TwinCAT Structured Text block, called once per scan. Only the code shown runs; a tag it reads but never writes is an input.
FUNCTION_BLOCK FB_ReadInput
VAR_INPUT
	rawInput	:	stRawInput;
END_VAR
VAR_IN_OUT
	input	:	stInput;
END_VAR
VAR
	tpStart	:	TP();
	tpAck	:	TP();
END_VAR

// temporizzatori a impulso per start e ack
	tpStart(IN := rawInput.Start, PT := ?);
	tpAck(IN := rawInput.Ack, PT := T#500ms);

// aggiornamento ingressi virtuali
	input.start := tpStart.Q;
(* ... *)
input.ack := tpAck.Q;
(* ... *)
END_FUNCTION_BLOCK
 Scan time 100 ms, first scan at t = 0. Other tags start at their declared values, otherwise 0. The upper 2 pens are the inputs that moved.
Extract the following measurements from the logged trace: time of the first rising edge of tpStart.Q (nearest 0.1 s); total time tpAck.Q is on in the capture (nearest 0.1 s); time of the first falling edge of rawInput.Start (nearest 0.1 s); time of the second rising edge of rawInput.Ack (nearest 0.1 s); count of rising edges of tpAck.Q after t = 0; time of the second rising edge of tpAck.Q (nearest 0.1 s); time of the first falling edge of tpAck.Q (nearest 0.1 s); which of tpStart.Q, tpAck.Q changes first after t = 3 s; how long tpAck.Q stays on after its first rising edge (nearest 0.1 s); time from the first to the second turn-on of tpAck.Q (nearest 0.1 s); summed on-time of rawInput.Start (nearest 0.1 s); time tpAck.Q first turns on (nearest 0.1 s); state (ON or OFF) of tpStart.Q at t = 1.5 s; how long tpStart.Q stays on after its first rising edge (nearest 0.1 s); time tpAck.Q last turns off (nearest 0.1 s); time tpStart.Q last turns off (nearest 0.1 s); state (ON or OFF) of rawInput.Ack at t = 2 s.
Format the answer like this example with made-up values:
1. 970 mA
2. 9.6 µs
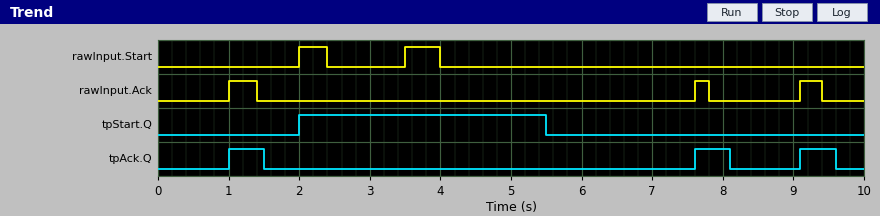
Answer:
1. 2.0 s
2. 1.5 s
3. 2.4 s
4. 7.6 s
5. 3
6. 7.6 s
7. 1.5 s
8. tpStart.Q
9. 0.5 s
10. 6.6 s
11. 0.9 s
12. 1.0 s
13. OFF
14. 3.5 s
15. 9.6 s
16. 5.5 s
17. OFF
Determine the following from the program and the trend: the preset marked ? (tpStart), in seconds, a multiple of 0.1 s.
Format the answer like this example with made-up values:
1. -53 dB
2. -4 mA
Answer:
1. 3.5 s
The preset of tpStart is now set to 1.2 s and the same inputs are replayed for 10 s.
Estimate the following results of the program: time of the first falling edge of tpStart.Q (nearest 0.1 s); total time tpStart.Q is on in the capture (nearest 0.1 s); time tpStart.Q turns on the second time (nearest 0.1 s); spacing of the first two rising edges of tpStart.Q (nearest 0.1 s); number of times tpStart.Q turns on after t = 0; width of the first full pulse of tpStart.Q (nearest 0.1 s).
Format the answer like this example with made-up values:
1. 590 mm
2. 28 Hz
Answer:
1. 3.2 s
2. 2.4 s
3. 3.5 s
4. 1.5 s
5. 2
6. 1.2 s
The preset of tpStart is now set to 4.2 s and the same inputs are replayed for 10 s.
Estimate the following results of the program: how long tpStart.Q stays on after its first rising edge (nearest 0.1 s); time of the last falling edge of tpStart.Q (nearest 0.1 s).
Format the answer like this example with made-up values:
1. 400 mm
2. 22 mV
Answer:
1. 4.2 s
2. 6.2 s
